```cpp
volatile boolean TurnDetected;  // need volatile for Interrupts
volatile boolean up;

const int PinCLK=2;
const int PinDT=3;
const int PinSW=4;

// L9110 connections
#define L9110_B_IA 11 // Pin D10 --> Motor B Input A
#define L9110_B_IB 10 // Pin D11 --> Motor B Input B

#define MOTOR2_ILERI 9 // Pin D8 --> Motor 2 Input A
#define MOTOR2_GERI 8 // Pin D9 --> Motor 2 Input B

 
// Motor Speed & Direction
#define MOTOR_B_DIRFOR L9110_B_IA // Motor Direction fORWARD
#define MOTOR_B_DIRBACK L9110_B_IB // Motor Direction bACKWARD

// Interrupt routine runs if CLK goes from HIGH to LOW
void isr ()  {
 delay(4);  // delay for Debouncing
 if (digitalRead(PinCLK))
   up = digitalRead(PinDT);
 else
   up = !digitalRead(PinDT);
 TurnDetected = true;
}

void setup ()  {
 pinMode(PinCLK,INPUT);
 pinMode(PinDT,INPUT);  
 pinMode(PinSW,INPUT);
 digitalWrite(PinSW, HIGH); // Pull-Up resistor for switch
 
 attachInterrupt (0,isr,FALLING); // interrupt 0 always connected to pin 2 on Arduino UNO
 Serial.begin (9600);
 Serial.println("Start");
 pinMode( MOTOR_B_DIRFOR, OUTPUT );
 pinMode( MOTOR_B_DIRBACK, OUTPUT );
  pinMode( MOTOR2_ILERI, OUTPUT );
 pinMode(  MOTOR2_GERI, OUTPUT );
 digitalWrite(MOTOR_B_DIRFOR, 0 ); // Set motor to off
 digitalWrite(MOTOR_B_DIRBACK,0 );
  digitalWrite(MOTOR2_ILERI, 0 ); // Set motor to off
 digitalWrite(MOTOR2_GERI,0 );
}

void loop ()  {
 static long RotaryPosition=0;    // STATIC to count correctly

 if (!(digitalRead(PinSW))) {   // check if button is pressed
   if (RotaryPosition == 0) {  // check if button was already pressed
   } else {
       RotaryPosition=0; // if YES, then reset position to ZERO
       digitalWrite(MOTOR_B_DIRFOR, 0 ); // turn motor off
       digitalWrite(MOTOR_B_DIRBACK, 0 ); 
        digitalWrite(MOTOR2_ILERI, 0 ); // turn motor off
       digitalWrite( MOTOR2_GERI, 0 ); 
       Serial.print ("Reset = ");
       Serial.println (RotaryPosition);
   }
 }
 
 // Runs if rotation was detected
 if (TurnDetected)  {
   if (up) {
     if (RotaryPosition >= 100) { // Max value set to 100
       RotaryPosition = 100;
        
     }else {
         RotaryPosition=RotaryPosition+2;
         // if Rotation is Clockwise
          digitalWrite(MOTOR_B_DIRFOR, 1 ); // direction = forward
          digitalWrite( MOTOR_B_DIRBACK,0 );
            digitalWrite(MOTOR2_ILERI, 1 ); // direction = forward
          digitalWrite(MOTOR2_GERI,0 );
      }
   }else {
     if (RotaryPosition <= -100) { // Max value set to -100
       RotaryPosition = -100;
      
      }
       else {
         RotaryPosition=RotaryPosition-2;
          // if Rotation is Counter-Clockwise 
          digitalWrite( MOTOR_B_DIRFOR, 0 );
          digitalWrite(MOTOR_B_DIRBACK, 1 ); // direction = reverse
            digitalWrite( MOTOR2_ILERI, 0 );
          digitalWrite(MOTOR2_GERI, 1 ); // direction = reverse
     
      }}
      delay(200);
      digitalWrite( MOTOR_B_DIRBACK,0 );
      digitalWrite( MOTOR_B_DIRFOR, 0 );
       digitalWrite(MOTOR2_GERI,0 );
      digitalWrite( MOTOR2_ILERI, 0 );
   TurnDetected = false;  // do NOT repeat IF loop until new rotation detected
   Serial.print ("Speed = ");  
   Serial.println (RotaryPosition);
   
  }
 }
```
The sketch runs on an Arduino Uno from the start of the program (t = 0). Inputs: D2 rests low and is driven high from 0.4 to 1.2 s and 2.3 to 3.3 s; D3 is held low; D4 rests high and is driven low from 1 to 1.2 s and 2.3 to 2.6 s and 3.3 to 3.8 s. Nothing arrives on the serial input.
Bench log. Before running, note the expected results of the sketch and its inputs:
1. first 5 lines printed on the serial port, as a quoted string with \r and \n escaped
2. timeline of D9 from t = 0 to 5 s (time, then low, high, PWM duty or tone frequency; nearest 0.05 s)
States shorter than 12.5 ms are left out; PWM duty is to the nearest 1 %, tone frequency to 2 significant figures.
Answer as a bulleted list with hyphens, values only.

- "Start\r\nSpeed = 2\r\nReset = 0\r\nSpeed = 2\r\nReset = 0\r\n"
- 0 s low; 1.2 s high; 1.4 s low; 3.3 s high; 3.5 s low
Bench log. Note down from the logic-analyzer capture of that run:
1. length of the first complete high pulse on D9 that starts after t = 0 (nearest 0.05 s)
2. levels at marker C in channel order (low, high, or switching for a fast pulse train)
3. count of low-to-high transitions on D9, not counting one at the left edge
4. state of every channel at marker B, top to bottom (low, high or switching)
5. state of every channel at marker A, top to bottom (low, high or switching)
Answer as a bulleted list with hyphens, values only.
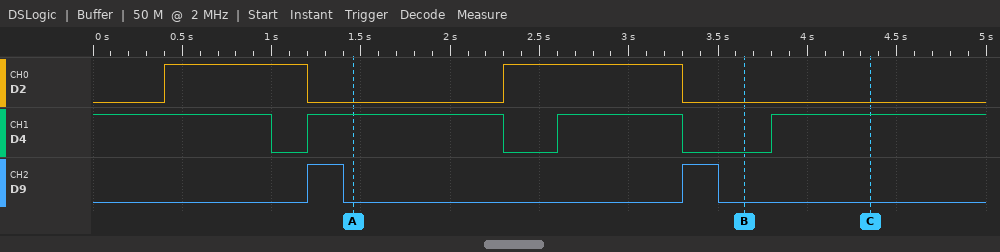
- 0.20 s
- D2 low, D4 high, D9 low
- 2
- D2 low, D4 low, D9 low
- D2 low, D4 high, D9 low
